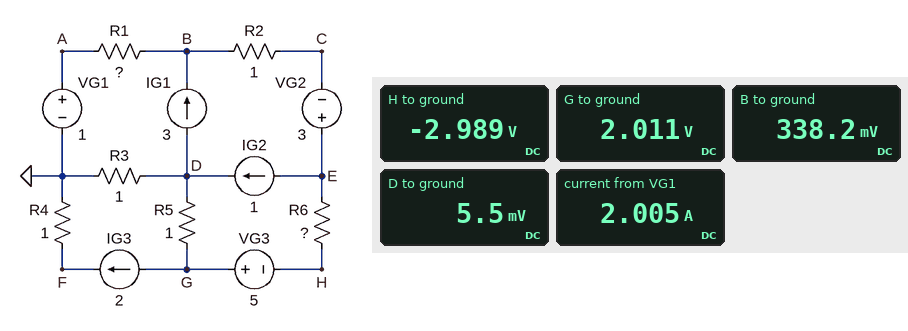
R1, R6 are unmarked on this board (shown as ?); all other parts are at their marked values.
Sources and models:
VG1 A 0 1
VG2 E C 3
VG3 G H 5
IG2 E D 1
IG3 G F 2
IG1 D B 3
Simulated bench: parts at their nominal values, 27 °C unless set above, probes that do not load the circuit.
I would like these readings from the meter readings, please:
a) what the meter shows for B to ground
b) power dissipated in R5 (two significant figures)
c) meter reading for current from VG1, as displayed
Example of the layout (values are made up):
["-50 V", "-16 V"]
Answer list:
["338.2 mV", "4.0 W", "2.005 A"]
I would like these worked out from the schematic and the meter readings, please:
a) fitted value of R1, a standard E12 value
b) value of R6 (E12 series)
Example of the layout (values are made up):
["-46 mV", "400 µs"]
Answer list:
["0.33 Ω", "0.33 Ω"]
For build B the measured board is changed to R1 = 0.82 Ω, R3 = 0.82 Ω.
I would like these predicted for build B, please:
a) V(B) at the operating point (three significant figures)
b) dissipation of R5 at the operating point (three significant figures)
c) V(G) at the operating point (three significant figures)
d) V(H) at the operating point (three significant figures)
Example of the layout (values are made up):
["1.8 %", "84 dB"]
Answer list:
["-442 mV", "3.09 W", "1.56 V", "-3.44 V"]
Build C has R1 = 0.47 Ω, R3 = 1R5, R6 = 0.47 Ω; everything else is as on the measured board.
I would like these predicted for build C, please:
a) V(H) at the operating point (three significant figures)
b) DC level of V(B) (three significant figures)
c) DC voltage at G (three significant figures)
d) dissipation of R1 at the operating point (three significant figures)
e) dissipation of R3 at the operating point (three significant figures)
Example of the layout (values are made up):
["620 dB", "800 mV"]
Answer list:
["-3.46 V", "147 mV", "1.54 V", "1.55 W", "51.2 mW"]
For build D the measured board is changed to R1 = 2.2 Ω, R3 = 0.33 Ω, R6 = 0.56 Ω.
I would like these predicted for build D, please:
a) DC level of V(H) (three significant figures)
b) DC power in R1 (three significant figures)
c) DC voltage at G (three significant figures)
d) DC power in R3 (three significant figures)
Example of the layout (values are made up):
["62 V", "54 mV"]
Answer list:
["-4.21 V", "2.61 W", "788 mV", "274 mW"]
